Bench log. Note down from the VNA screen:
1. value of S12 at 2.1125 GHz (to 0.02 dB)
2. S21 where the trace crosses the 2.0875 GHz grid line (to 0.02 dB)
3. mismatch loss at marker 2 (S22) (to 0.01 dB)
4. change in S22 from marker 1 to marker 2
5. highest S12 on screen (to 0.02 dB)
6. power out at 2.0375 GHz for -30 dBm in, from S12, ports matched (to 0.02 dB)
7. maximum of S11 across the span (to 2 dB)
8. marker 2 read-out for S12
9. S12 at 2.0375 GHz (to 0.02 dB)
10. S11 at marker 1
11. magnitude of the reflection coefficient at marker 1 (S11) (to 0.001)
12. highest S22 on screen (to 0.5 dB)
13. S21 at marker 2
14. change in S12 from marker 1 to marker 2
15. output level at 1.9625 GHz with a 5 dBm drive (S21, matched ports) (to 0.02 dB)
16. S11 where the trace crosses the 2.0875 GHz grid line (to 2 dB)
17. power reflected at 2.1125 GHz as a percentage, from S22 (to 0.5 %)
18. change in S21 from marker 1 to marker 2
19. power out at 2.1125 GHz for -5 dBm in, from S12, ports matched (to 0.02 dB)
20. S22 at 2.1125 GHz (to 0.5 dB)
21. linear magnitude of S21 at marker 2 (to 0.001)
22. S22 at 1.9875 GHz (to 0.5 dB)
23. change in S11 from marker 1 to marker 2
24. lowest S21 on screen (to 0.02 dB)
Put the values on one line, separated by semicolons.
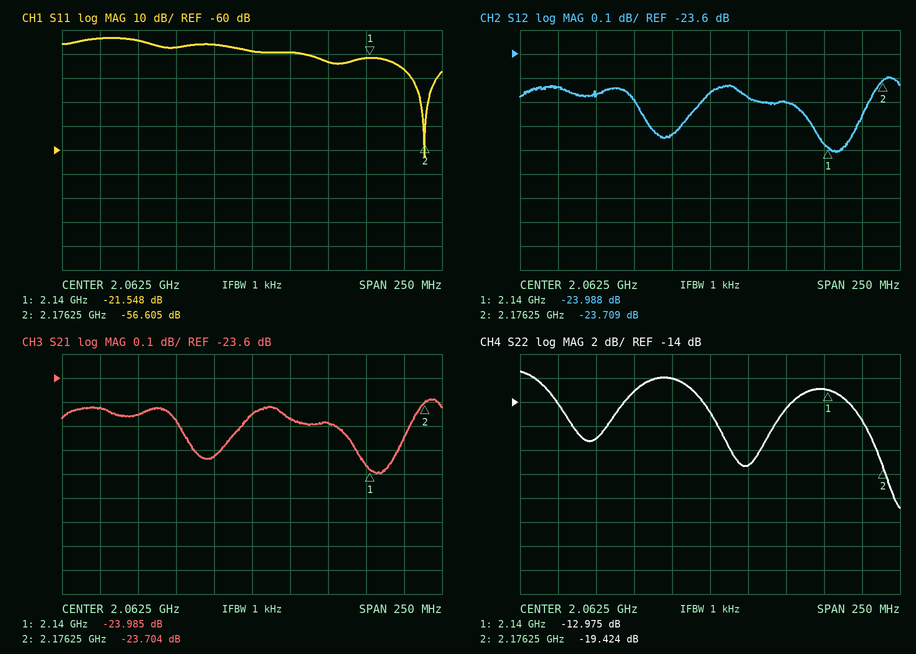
-23.80 dB; -23.76 dB; 0.05 dB; -6.449 dB; -23.70 dB; -53.94 dBm; -14 dB; -23.709 dB; -23.94 dB; -21.548 dB; 0.084; -11.5 dB; -23.704 dB; 0.279 dB; -18.72 dBm; -20 dB; 3.5 %; 0.281 dB; -28.80 dBm; -14.5 dB; 0.065; -17.0 dB; -35.057 dB; -24.00 dB
